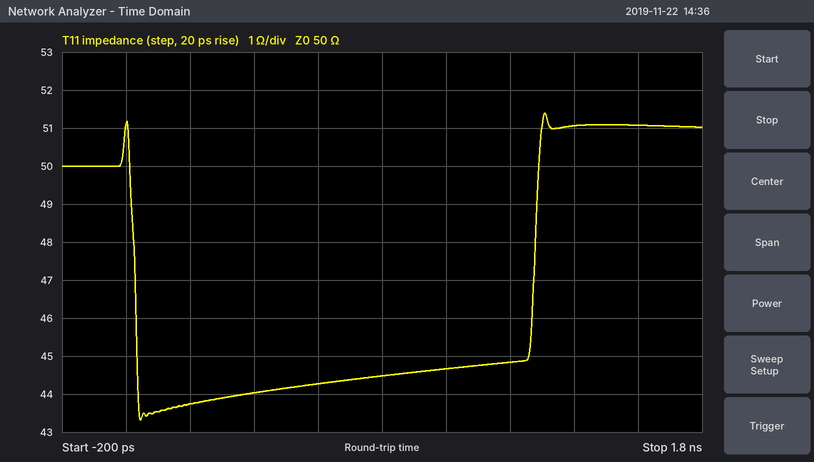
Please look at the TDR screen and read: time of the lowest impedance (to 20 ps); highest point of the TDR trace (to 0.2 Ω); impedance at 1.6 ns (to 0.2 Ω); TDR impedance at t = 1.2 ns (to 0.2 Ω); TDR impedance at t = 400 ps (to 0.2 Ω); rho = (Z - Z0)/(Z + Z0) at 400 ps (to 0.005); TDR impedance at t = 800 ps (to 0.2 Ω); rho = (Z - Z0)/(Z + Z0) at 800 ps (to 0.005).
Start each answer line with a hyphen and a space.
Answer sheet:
- 40 ps
- 51.4 Ω
- 51.0 Ω
- 44.8 Ω
- 44.0 Ω
- -0.065
- 44.4 Ω
- -0.060
